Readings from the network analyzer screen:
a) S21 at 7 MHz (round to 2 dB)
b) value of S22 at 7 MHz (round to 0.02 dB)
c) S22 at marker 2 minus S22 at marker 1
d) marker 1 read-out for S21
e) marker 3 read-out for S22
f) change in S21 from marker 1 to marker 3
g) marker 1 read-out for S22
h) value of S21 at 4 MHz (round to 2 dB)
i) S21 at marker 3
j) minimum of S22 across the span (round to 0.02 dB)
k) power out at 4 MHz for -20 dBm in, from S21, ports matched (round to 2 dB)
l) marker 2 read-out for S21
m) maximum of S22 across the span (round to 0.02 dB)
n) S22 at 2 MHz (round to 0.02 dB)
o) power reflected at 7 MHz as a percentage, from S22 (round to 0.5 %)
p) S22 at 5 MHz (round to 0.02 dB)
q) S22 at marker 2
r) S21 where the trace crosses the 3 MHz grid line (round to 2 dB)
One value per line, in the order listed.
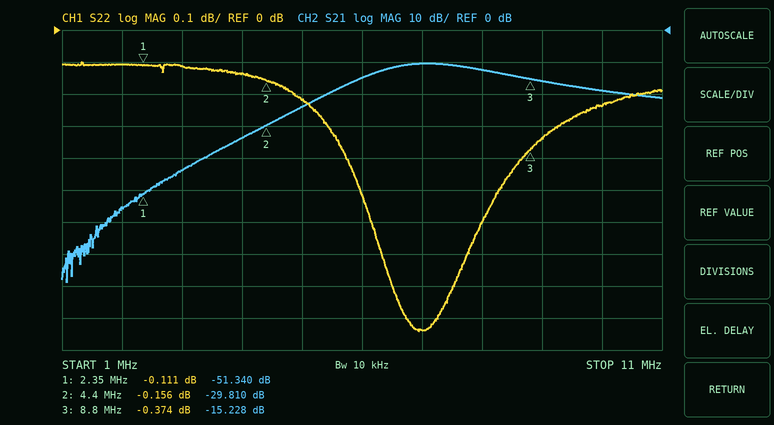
-10 dB
-0.94 dB
-0.045 dB
-51.340 dB
-0.374 dB
36.112 dB
-0.111 dB
-34 dB
-15.228 dB
-0.94 dB
-54 dBm
-29.810 dB
-0.10 dB
-0.10 dB
80.5 %
-0.22 dB
-0.156 dB
-44 dB
